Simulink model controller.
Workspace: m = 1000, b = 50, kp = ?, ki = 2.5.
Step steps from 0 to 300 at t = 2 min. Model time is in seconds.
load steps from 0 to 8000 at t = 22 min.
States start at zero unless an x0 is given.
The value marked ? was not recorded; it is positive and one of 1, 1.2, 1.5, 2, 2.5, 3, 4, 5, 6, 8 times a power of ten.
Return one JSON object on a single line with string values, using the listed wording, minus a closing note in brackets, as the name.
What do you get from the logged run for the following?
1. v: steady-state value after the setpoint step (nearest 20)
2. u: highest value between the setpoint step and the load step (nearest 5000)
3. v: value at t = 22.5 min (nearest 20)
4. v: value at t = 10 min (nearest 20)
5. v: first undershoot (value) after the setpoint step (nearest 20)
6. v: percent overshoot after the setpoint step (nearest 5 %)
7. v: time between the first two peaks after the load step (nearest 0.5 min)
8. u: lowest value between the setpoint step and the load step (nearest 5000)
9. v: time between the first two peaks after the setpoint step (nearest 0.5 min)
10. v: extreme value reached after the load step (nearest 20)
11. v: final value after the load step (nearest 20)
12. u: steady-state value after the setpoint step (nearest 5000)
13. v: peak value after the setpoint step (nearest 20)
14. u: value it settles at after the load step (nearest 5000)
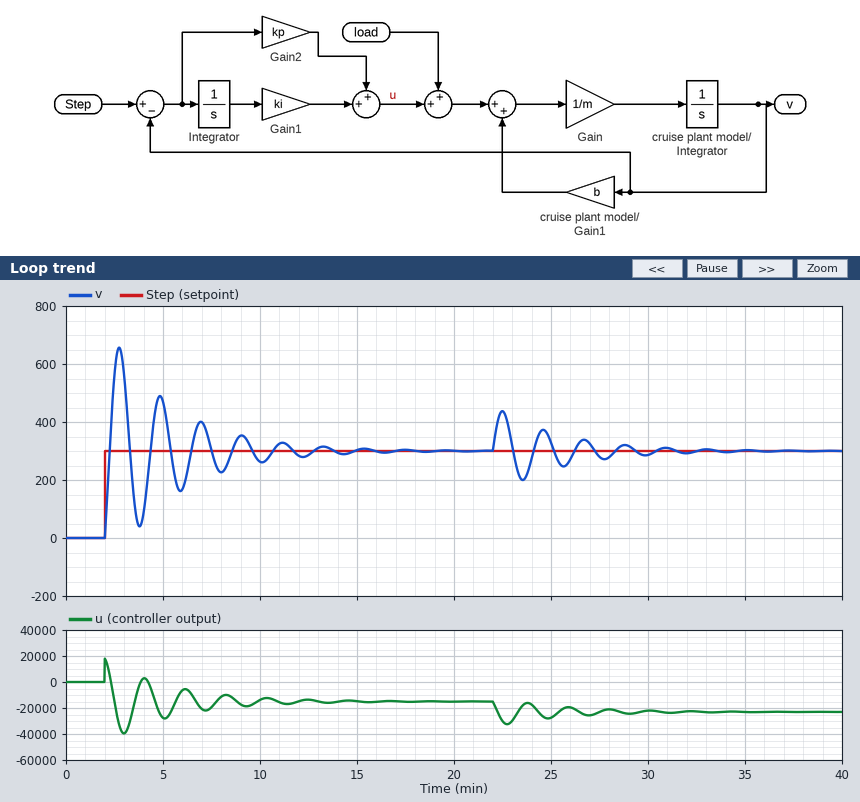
{"v: steady-state value after the setpoint step": "300", "u: highest value between the setpoint step and the load step": "20000", "v: value at t = 22.5 min": "440", "v: value at t = 10 min": "260", "v: first undershoot (value) after the setpoint step": "40", "v: percent overshoot after the setpoint step": "120 %", "v: time between the first two peaks after the load step": "2.0 min", "u: lowest value between the setpoint step and the load step": "-40000", "v: time between the first two peaks after the setpoint step": "2.0 min", "v: extreme value reached after the load step": "440", "v: final value after the load step": "300", "u: steady-state value after the setpoint step": "-15000", "v: peak value after the setpoint step": "660", "u: value it settles at after the load step": "-25000"}
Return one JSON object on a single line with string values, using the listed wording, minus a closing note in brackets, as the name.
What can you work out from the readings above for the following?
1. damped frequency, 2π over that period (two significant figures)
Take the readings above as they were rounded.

{"damped frequency, 2π over that period": "3.1 rad/min"}
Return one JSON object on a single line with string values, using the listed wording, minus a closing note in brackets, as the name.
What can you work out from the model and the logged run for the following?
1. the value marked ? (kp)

{"the value marked ?": "60"}
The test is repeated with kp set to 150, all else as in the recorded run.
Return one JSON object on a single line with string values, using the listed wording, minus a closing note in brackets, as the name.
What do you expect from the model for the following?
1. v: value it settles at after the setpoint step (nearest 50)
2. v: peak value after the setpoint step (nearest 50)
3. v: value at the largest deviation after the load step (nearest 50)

{"v: value it settles at after the setpoint step": "300", "v: peak value after the setpoint step": "450", "v: value at the largest deviation after the load step": "350"}
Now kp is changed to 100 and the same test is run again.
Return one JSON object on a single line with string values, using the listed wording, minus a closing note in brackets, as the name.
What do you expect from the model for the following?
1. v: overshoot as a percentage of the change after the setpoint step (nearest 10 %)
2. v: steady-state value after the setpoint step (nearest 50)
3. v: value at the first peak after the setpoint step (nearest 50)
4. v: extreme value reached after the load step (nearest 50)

{"v: overshoot as a percentage of the change after the setpoint step": "70 %", "v: steady-state value after the setpoint step": "300", "v: value at the first peak after the setpoint step": "500", "v: extreme value reached after the load step": "400"}
